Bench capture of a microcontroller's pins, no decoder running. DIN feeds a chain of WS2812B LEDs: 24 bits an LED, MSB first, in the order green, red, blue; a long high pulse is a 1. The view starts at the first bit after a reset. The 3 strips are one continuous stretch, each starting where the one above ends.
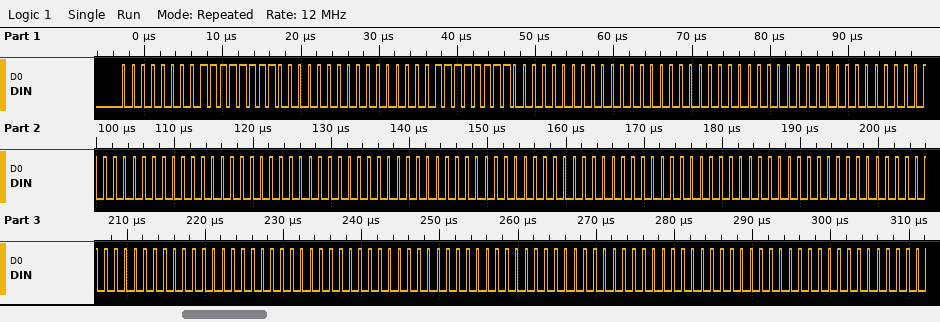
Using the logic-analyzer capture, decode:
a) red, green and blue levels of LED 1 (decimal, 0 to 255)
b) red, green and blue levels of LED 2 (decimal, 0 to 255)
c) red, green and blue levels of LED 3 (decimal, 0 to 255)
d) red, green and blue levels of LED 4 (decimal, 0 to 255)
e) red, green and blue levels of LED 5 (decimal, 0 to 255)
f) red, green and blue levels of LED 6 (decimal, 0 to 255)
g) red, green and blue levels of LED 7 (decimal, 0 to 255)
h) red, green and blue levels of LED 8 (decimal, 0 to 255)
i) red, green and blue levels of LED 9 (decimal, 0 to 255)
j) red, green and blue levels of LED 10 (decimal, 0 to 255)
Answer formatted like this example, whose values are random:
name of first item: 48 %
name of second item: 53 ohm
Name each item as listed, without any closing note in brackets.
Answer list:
red, green and blue levels of LED 1: 255, 0, 0
red, green and blue levels of LED 2: 255, 0, 0
red, green and blue levels of LED 3: 0, 0, 0
red, green and blue levels of LED 4: 0, 0, 0
red, green and blue levels of LED 5: 0, 0, 0
red, green and blue levels of LED 6: 0, 0, 0
red, green and blue levels of LED 7: 0, 0, 0
red, green and blue levels of LED 8: 0, 0, 0
red, green and blue levels of LED 9: 0, 0, 0
red, green and blue levels of LED 10: 0, 0, 0
